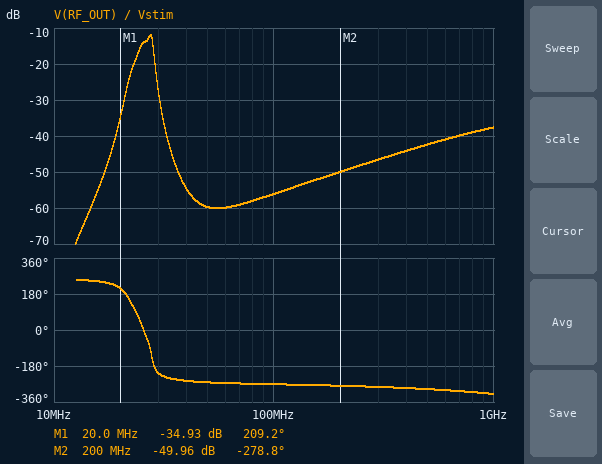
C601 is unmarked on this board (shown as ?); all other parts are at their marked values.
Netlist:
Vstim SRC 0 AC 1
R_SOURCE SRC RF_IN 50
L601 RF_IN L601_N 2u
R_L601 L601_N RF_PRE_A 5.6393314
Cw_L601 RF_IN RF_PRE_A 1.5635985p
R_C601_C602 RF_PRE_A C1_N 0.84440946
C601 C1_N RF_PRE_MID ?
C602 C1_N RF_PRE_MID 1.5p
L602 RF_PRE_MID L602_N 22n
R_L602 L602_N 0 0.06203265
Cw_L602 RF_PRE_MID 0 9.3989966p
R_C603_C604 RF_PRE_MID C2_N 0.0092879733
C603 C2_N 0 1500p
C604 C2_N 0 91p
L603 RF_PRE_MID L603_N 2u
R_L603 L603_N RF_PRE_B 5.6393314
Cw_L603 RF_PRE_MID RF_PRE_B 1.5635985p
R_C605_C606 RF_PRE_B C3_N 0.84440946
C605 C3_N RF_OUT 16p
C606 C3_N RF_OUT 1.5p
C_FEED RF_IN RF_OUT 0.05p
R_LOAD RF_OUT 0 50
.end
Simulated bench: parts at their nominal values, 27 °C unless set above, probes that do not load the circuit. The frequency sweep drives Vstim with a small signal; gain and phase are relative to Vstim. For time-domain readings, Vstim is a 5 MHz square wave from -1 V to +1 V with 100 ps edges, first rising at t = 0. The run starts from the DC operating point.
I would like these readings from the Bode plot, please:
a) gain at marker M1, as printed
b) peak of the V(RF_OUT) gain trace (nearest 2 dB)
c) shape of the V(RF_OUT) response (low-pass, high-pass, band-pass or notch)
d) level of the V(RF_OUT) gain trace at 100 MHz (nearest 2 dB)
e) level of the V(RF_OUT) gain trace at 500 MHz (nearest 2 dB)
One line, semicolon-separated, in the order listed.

-34.93 dB; -12 dB; band-pass; -56 dB; -42 dB
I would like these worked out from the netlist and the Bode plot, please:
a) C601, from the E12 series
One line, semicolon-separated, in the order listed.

22 pF
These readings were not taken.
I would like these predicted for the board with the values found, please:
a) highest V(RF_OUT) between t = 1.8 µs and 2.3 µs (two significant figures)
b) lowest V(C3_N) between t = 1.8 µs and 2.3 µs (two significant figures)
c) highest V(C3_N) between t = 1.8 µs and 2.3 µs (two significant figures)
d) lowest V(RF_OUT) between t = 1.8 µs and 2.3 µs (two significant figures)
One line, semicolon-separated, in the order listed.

48 mV; -350 mV; 350 mV; -48 mV
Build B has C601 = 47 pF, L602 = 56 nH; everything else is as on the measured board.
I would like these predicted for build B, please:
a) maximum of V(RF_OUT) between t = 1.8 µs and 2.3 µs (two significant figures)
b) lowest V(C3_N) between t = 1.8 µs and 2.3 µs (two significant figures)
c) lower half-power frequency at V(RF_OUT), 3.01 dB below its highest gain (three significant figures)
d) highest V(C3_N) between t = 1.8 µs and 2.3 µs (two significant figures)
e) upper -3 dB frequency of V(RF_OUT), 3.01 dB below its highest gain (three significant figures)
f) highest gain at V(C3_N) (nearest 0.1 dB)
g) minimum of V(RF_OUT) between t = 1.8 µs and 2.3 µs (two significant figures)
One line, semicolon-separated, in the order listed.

30 mV; -340 mV; 16.3 MHz; 340 mV; 18.0 MHz; 4.2 dB; -30 mV
